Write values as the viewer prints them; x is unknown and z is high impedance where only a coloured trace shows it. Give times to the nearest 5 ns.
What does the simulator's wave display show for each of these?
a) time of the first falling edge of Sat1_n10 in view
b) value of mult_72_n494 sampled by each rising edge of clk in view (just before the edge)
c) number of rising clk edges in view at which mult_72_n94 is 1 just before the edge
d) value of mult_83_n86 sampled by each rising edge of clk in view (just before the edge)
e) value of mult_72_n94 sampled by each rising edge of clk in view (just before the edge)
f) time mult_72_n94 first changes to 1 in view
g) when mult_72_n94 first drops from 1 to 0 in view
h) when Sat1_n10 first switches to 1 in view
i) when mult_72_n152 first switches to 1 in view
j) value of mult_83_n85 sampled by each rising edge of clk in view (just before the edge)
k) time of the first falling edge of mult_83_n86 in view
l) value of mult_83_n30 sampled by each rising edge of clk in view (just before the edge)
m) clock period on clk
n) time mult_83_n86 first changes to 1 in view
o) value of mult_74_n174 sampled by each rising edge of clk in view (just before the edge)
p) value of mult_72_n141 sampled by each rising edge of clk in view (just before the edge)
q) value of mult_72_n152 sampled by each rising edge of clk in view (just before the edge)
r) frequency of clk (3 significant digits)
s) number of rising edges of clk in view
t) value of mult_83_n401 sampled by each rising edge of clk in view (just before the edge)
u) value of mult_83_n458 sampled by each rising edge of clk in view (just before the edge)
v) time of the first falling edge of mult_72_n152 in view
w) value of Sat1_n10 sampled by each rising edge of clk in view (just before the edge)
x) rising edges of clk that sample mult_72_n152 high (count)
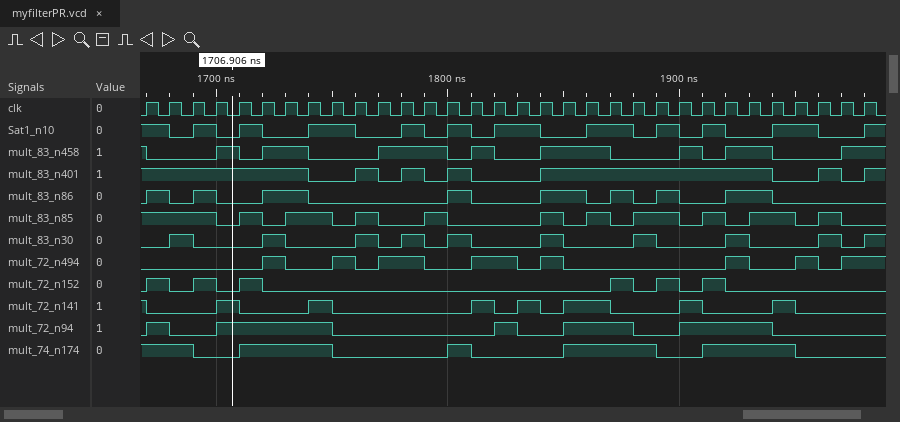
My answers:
1680 ns
0 0 0 0 0 0 1 0 0 1 0 1 1 0 0 1 1 0 1 0 0 0 0 0 0 0 1 0 0 1 0 1
14
0 1 0 1 0 0 1 1 0 0 0 0 0 0 1 0 0 0 1 1 0 1 0 1 0 0 1 1 0 0 0 0
0 1 0 0 1 1 1 1 1 0 0 0 0 0 0 0 1 0 0 1 1 1 0 0 1 1 1 1 0 0 0 0
1670 ns
1680 ns
1690 ns
1670 ns
1 1 1 1 0 1 0 1 1 0 1 0 0 1 0 0 0 0 1 0 1 0 1 1 0 1 0 1 1 0 1 0
1680 ns
0 0 1 0 0 0 1 0 0 0 1 0 1 0 1 0 0 0 1 0 0 0 1 0 0 0 1 0 0 0 1 0
10 ns
1670 ns
1 1 1 0 0 1 1 1 1 0 0 0 0 0 1 0 0 0 0 1 1 1 1 0 0 1 1 1 1 0 0 0
1 0 0 0 1 0 0 0 1 0 0 0 0 0 0 1 0 1 0 1 1 0 0 0 1 0 0 0 1 0 0 0
0 1 0 1 0 1 0 0 0 0 0 0 0 0 0 0 0 0 0 0 0 1 0 1 0 1 0 0 0 0 0 0
100 MHz
32
1 1 1 1 1 1 1 1 0 0 1 0 1 0 1 0 0 0 1 1 1 1 1 1 1 1 1 1 0 0 1 0
1 0 0 0 1 0 1 1 0 0 0 1 1 1 0 1 0 0 1 1 1 0 0 0 1 0 1 1 0 0 0 1
1680 ns
1 1 0 1 0 1 0 0 1 1 0 0 1 0 1 0 1 1 0 0 1 1 0 1 0 1 0 0 1 1 0 0
6
